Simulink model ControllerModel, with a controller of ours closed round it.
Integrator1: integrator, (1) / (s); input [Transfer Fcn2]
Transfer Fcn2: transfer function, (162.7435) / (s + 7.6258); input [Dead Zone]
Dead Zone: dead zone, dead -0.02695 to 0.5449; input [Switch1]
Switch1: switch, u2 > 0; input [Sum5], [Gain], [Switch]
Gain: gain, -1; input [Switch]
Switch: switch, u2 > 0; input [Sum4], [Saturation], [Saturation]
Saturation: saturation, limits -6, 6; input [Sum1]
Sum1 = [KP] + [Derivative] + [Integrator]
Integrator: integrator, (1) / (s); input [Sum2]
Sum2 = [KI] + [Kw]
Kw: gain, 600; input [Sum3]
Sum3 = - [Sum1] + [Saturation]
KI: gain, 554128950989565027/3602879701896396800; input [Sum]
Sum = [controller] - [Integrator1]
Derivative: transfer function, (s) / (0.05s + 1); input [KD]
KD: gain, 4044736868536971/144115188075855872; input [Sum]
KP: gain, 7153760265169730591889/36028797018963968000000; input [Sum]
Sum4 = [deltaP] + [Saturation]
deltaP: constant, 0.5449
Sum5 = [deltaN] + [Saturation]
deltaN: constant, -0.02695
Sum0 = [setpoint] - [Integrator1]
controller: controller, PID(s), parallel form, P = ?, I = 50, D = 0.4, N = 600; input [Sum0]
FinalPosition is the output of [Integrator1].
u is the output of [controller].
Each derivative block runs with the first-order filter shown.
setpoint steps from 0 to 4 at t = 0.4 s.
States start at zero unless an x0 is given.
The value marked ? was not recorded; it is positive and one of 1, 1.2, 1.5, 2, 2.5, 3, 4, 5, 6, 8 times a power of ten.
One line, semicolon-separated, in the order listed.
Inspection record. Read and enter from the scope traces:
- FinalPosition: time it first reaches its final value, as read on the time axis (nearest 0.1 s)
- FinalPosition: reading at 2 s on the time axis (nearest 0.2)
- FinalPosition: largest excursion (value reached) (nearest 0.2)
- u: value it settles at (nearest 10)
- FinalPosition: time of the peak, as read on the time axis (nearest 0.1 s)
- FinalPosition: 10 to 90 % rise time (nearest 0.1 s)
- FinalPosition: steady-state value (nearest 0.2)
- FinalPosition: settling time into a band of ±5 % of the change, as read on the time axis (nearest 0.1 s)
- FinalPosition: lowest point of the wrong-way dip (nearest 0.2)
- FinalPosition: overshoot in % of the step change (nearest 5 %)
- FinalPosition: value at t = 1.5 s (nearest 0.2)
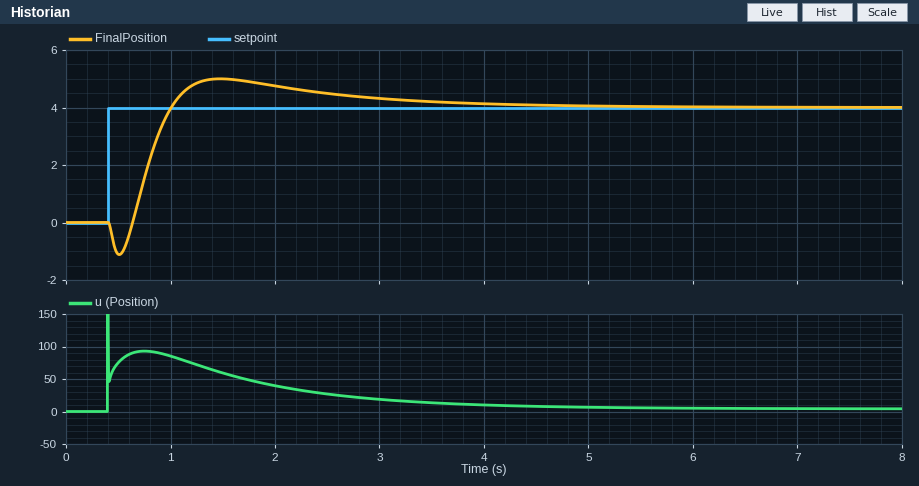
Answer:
1.0 s; 4.8; 5.0; 0; 1.5 s; 0.3 s; 4.0; 3.5 s; -1.2; 25 %; 5.0
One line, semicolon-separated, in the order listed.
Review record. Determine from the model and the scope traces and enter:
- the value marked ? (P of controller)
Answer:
10
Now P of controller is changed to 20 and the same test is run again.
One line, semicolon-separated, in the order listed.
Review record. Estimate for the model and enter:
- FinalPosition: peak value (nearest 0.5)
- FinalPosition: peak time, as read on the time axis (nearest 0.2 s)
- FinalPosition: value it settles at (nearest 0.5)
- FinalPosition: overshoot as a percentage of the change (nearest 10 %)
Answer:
5.5; 2.0 s; 4.0; 40 %
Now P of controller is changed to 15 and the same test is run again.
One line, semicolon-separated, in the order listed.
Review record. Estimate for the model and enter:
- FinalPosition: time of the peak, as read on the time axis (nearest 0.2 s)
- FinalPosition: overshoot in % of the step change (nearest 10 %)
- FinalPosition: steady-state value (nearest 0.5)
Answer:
1.8 s; 30 %; 4.0
